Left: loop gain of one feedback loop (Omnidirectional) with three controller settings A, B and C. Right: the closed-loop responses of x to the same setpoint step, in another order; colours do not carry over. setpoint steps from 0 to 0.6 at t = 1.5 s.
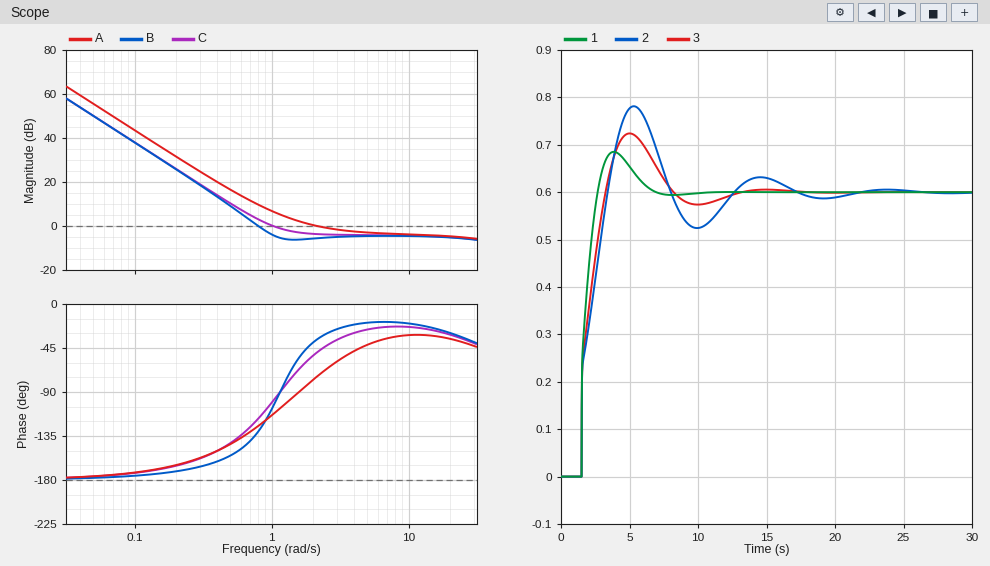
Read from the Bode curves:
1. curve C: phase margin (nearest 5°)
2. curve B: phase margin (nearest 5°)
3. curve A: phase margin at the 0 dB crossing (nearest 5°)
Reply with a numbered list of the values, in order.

1. 80°
2. 50°
3. 105°
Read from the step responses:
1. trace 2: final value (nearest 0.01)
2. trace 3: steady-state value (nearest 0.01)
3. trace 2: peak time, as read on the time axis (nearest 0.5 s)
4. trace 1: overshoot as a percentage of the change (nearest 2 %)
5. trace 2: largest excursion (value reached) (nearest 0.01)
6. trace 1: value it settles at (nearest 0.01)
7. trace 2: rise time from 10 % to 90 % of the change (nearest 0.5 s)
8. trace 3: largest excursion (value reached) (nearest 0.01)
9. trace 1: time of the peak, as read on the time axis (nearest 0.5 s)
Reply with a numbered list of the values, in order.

1. 0.60
2. 0.60
3. 5.5 s
4. 14 %
5. 0.78
6. 0.60
7. 1.5 s
8. 0.72
9. 4.0 s
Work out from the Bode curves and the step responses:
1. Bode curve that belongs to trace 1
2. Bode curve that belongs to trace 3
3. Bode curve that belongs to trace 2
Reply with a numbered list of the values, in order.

1. A
2. C
3. B
